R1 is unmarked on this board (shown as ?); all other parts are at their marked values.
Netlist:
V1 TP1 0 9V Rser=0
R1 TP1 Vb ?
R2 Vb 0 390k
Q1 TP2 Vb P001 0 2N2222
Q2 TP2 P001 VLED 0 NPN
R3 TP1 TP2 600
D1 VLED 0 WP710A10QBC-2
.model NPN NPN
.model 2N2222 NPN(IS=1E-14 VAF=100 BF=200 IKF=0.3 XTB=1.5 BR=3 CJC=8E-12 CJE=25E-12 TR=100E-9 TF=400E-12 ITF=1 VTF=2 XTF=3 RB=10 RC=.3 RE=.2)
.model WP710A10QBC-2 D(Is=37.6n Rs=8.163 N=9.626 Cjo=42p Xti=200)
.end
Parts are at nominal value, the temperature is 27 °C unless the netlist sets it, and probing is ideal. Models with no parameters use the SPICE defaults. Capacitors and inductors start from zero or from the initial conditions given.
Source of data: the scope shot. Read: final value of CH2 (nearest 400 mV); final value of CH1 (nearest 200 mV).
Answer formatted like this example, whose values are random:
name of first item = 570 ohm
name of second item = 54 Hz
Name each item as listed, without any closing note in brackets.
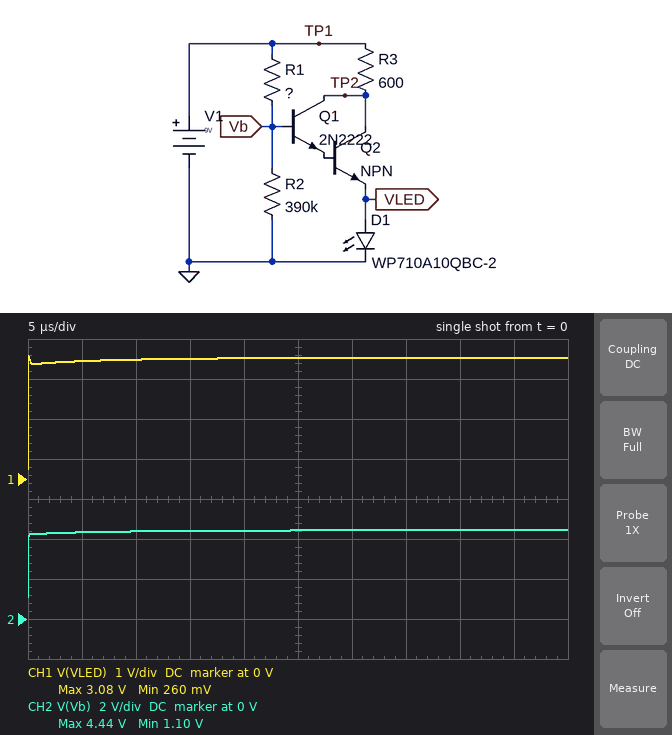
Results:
final value of CH2 = 4.4 V
final value of CH1 = 3.0 V
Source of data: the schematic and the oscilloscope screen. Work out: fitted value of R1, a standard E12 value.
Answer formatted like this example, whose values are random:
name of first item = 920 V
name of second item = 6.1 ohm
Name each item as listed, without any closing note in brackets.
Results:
fitted value of R1, a standard E12 value = 390 kΩ
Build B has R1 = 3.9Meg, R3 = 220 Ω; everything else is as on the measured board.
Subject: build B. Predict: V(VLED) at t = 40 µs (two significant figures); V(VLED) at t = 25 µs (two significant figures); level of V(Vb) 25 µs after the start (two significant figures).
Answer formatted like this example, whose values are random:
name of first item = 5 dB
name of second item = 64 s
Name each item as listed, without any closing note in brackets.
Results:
V(VLED) at t = 40 µs = 670 mV
V(VLED) at t = 25 µs = 820 mV
level of V(Vb) 25 µs after the start = 830 mV
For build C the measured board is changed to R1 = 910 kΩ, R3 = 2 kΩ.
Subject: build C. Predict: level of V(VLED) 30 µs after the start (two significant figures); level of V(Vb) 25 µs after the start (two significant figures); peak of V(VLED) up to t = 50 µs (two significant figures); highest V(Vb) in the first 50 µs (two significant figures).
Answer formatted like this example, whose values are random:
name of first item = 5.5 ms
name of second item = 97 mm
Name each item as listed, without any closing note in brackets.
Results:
level of V(VLED) 30 µs after the start = 1.6 V
level of V(Vb) 25 µs after the start = 2.7 V
peak of V(VLED) up to t = 50 µs = 2.8 V
highest V(Vb) in the first 50 µs = 3.9 V
